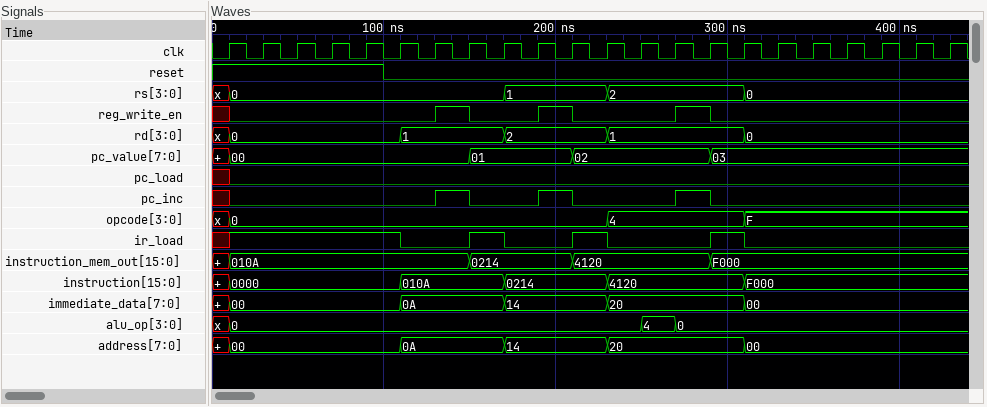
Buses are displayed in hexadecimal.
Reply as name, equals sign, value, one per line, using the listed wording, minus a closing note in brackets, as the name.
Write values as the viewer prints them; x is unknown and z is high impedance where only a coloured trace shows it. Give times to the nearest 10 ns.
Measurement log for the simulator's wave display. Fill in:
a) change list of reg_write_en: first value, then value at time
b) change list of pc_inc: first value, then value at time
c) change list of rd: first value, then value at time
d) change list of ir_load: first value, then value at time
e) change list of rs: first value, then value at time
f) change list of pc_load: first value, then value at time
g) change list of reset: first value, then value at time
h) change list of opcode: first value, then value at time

change list of reg_write_en: first value, then value at time = x, 0 at 10 ns, 1 at 130 ns, 0 at 150 ns, 1 at 190 ns, 0 at 210 ns, 1 at 270 ns, 0 at 290 ns
change list of pc_inc: first value, then value at time = x, 0 at 10 ns, 1 at 130 ns, 0 at 150 ns, 1 at 190 ns, 0 at 210 ns, 1 at 270 ns, 0 at 290 ns
change list of rd: first value, then value at time = x, 0 at 10 ns, 1 at 110 ns, 2 at 170 ns, 1 at 230 ns, 0 at 310 ns
change list of ir_load: first value, then value at time = x, 1 at 10 ns, 0 at 110 ns, 1 at 150 ns, 0 at 170 ns, 1 at 210 ns, 0 at 230 ns, 1 at 290 ns, 0 at 310 ns
change list of rs: first value, then value at time = x, 0 at 10 ns, 1 at 170 ns, 2 at 230 ns, 0 at 310 ns
change list of pc_load: first value, then value at time = x, 0 at 10 ns
change list of reset: first value, then value at time = 1, 0 at 100 ns
change list of opcode: first value, then value at time = x, 0 at 10 ns, 4 at 230 ns, F at 310 ns
